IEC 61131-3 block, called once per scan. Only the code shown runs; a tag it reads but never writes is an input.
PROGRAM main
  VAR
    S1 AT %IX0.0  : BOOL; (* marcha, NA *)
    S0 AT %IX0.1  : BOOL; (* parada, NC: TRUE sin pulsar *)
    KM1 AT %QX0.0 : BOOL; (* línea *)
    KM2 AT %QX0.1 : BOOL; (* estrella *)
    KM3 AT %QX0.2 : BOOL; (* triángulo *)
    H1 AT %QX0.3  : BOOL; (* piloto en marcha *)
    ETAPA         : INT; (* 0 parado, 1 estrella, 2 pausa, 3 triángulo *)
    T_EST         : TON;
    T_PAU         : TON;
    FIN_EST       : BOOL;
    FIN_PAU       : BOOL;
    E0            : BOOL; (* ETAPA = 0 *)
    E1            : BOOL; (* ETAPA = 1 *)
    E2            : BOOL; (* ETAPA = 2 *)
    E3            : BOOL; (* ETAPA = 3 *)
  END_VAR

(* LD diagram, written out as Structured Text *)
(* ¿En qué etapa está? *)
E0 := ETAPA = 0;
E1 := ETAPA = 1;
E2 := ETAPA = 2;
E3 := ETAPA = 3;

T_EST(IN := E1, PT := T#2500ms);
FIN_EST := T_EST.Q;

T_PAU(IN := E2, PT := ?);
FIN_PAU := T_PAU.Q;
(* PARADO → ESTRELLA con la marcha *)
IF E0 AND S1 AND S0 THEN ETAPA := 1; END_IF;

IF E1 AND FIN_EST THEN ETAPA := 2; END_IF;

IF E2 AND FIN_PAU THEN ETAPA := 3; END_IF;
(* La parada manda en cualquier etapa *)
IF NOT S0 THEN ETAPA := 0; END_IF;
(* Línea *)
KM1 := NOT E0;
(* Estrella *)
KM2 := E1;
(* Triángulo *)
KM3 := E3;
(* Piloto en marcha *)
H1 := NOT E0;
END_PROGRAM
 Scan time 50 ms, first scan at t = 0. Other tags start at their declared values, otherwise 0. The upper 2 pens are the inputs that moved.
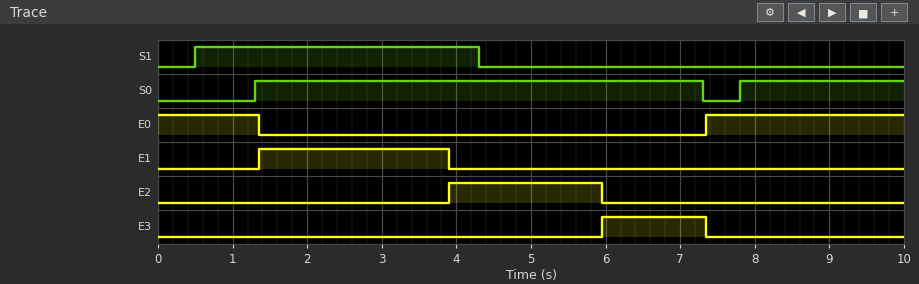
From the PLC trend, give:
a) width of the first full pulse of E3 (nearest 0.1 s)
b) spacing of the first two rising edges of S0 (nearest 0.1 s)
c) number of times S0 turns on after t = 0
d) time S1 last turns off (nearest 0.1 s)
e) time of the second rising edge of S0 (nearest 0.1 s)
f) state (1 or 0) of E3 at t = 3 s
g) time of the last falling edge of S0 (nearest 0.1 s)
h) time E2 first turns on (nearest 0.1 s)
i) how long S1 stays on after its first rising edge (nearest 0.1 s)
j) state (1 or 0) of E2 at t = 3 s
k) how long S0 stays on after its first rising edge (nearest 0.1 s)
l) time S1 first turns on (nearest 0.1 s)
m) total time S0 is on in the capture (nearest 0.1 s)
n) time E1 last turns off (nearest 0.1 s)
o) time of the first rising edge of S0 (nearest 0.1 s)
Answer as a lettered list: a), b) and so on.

a) 1.4 s
b) 6.5 s
c) 2
d) 4.3 s
e) 7.8 s
f) 0
g) 7.3 s
h) 3.9 s
i) 3.8 s
j) 0
k) 6.0 s
l) 0.5 s
m) 8.2 s
n) 3.9 s
o) 1.3 s
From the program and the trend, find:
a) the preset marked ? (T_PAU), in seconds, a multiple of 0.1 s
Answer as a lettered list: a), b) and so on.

a) 2.0 s
